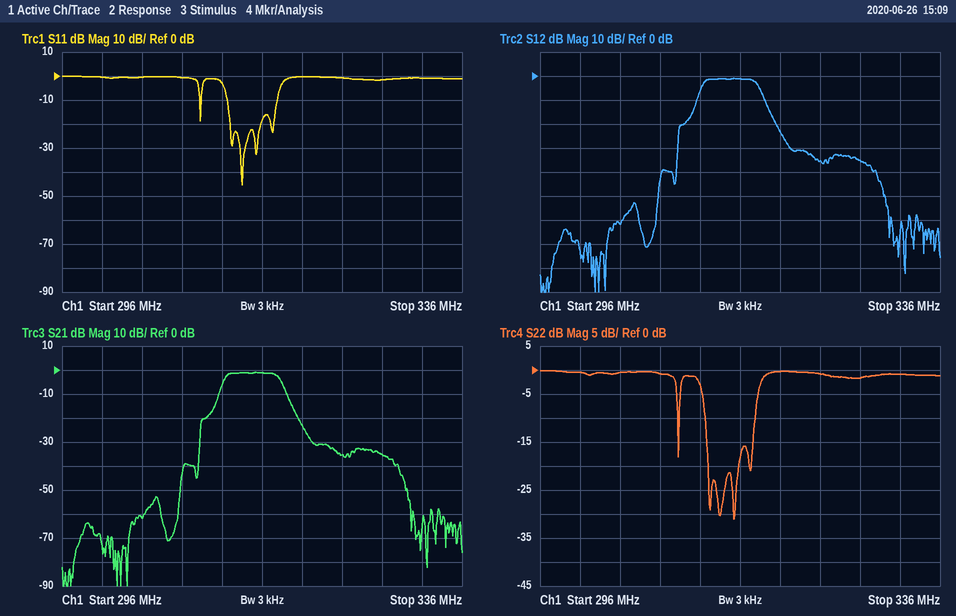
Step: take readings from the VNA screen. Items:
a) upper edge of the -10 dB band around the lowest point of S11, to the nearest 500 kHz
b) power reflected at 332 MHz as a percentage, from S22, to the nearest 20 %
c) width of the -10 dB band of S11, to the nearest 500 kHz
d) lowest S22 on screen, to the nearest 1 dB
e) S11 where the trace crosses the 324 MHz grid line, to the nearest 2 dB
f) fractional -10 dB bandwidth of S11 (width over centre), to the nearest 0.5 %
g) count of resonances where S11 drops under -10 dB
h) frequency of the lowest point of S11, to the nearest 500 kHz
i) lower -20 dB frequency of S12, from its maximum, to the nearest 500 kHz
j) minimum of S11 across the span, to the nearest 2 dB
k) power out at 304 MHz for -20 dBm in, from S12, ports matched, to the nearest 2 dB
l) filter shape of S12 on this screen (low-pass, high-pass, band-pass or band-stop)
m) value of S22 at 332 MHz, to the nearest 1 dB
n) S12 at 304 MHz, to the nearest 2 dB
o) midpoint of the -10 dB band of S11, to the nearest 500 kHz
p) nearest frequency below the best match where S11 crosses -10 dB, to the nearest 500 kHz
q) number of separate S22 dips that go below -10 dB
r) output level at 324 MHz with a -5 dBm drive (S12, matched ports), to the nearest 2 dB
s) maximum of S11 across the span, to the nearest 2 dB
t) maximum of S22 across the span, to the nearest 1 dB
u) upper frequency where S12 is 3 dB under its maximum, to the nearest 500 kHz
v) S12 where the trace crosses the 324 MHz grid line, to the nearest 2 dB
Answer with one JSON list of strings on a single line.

["317.5 MHz", "80 %", "5.0 MHz", "-31 dB", "0 dB", "1.5 %", "5", "314.0 MHz", "310.0 MHz", "-46 dB", "-82 dBm", "band-pass", "-1 dB", "-62 dB", "315.0 MHz", "312.5 MHz", "5", "-40 dBm", "0 dB", "0 dB", "318.0 MHz", "-36 dB"]
